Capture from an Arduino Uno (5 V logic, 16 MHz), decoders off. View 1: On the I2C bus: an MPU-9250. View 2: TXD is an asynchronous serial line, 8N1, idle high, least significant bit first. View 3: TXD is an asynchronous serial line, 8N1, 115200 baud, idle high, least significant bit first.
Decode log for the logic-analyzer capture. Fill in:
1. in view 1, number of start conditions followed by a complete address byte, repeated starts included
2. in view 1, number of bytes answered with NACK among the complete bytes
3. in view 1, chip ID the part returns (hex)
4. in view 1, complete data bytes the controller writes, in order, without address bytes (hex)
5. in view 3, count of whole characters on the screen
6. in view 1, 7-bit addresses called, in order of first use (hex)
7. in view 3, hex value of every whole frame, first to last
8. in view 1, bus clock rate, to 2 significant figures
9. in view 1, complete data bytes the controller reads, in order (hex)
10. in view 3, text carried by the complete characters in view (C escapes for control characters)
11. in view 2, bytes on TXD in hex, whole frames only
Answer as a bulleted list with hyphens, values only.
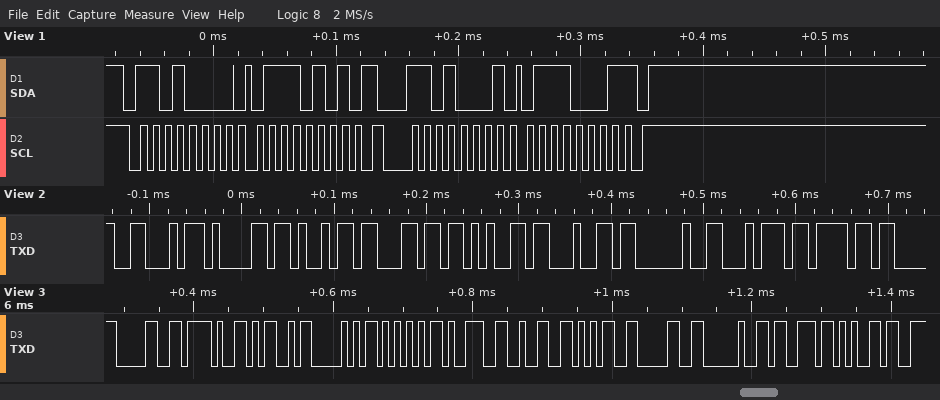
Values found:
- 2
- 1
- 0x71
- 75
- 12
- 0x68
- 30 2F 4D 50 55 39 32 35 30 20 73 65
- 100 kHz
- 71
- "0/MPU9250 se"
- 0x46 0x61 0x69 0x6C 0x65 0x64 0x20 0x74 0x6F
